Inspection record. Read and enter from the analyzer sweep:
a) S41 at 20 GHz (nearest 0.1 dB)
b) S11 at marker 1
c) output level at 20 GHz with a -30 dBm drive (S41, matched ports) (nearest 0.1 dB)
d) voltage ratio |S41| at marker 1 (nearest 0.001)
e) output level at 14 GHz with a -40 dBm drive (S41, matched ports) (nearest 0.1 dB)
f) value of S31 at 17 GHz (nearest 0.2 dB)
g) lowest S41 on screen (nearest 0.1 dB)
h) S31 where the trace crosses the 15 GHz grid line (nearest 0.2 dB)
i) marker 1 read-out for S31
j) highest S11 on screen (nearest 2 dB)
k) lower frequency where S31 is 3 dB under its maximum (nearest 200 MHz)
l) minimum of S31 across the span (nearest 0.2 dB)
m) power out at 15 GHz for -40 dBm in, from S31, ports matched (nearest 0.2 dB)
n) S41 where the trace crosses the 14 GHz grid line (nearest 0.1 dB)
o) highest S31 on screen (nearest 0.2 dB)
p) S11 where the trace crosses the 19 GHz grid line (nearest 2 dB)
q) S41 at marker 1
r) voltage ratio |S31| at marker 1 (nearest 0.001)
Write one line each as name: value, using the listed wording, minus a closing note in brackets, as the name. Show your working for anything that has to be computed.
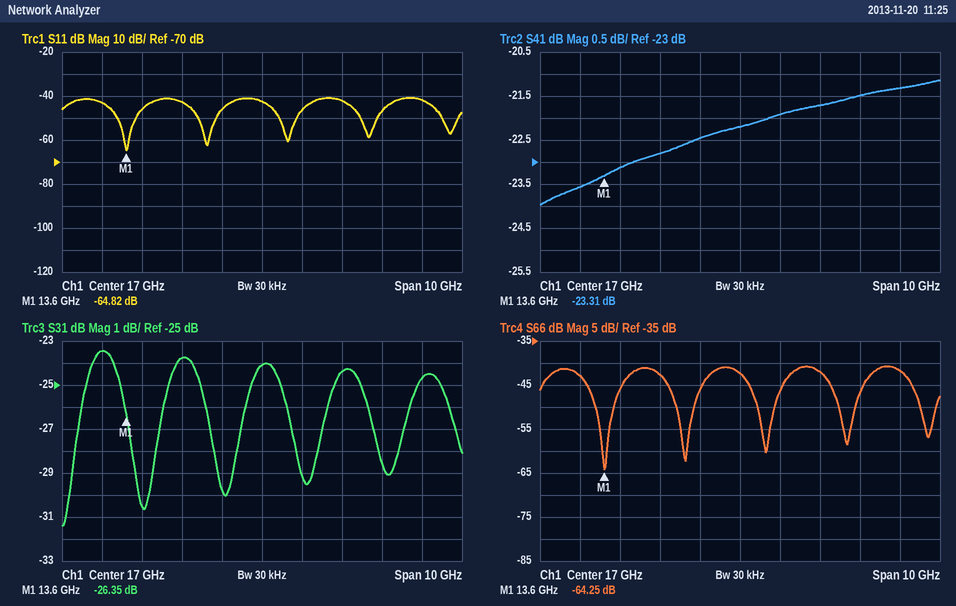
S41 at 20 GHz: -21.5 dB
S11 at marker 1: -64.82 dB
output level at 20 GHz with a -30 dBm drive (S41, matched ports): -30 dBm + (-21.5 dB) = -51.5 dBm
voltage ratio |S41| at marker 1: 10^(-23.31/20) ≈ 0.068
output level at 14 GHz with a -40 dBm drive (S41, matched ports): -40 dBm + (-23.1 dB) = -63.1 dBm
value of S31 at 17 GHz: -24.0 dB
lowest S41 on screen: -24.0 dB
S31 where the trace crosses the 15 GHz grid line: -23.8 dB
marker 1 read-out for S31: -26.35 dB
highest S11 on screen: -40 dB
lower frequency where S31 is 3 dB under its maximum: 12.4 GHz
minimum of S31 across the span: -31.4 dB
power out at 15 GHz for -40 dBm in, from S31, ports matched: -40 dBm + (-23.8 dB) = -63.8 dBm
S41 where the trace crosses the 14 GHz grid line: -23.1 dB
highest S31 on screen: -23.4 dB
S11 where the trace crosses the 19 GHz grid line: -42 dB
S41 at marker 1: -23.31 dB
voltage ratio |S31| at marker 1: 10^(-26.35/20) ≈ 0.048
